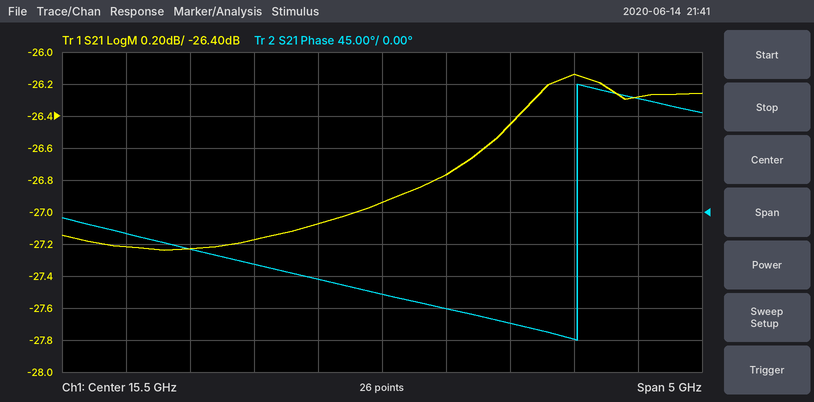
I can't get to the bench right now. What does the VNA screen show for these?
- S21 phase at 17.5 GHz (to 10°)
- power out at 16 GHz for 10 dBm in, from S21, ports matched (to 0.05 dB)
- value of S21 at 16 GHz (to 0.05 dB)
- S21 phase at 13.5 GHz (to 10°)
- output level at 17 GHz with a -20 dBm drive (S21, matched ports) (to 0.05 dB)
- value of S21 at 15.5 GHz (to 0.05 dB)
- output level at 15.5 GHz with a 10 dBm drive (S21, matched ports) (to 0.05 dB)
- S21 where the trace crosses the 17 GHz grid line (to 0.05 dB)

160°
-16.75 dBm
-26.75 dB
-30°
-46.15 dBm
-26.95 dB
-16.95 dBm
-26.15 dB
